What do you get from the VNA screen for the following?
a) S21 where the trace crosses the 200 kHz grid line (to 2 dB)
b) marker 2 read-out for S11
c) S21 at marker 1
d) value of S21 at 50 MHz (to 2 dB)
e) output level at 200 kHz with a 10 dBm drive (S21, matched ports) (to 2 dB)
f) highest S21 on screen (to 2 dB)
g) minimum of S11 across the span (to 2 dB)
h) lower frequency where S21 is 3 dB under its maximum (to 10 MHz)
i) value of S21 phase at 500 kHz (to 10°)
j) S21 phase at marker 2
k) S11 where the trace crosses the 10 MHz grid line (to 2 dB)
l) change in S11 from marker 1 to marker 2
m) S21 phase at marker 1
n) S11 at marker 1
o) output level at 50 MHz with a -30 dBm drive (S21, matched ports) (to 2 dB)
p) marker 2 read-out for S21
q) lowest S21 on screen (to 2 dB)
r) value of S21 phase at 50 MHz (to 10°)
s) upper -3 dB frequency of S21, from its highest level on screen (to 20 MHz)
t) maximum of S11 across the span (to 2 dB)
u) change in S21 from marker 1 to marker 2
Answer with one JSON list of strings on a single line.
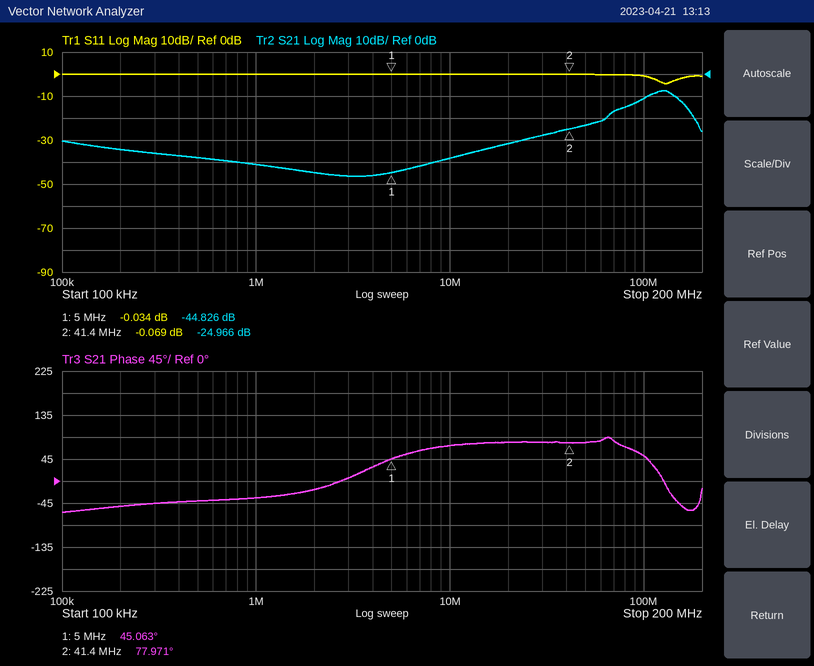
["-34 dB", "-0.069 dB", "-44.826 dB", "-24 dB", "-24 dBm", "-8 dB", "-4 dB", "100 MHz", "-40°", "77.971°", "0 dB", "-0.035 dB", "45.063°", "-0.034 dB", "-54 dBm", "-24.966 dB", "-46 dB", "80°", "140 MHz", "0 dB", "19.860 dB"]
